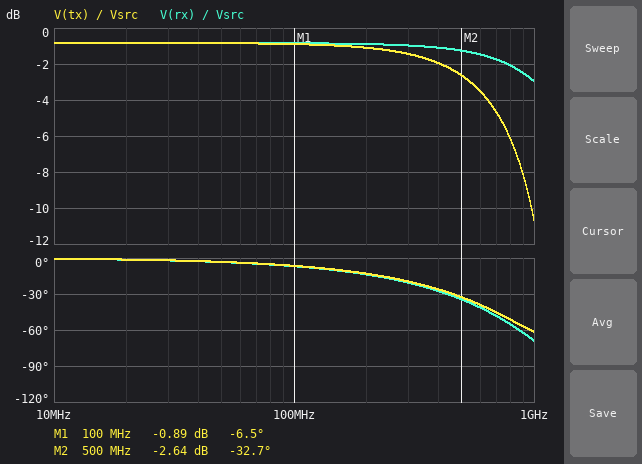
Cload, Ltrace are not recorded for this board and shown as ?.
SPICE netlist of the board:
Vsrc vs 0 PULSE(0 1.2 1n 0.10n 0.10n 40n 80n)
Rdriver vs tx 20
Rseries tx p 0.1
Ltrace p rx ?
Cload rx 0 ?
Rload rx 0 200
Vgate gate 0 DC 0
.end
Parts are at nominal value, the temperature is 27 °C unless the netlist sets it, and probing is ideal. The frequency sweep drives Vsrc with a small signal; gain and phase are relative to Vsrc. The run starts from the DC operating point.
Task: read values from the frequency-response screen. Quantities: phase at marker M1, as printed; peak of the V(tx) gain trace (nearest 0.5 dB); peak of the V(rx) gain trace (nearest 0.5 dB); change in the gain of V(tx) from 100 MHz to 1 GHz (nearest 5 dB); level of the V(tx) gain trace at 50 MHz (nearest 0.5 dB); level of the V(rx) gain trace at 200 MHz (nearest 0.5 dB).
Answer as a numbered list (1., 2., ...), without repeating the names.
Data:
1. -6.5 deg
2. -1.0 dB
3. -1.0 dB
4. -10 dB
5. -1.0 dB
6. -1.0 dB
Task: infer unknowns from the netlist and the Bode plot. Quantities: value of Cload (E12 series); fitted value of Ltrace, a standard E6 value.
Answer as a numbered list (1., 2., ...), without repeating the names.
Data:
1. 10 pF
2. 1.5 nH
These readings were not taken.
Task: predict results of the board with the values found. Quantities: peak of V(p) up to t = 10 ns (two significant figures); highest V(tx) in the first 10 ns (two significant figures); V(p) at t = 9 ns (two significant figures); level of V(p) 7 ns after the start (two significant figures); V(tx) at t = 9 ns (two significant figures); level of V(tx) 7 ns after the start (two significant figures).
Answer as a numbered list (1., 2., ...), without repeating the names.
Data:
1. 1.1 V
2. 1.1 V
3. 1.1 V
4. 1.1 V
5. 1.1 V
6. 1.1 V
